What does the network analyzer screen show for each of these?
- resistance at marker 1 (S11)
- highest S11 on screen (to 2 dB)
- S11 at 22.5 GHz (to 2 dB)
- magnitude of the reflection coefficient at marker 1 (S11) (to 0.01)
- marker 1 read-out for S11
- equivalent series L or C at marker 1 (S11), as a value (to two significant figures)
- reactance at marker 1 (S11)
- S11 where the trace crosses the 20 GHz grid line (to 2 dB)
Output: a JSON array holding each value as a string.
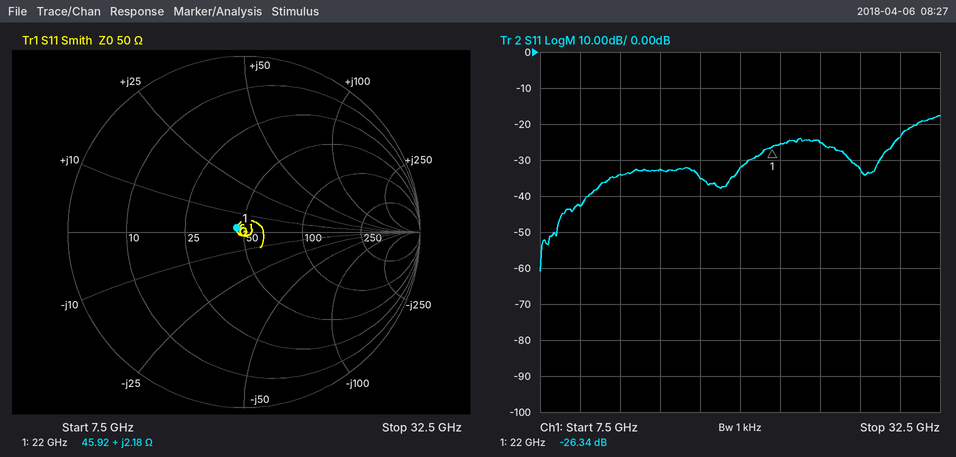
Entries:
["45.92 Ω", "-18 dB", "-26 dB", "0.05", "-26.34 dB", "16 pH", "+2.18 Ω", "-32 dB"]
